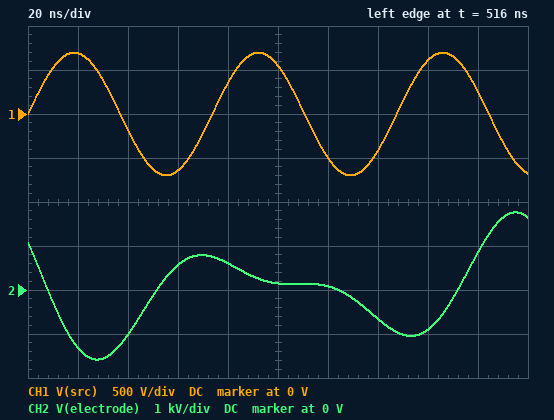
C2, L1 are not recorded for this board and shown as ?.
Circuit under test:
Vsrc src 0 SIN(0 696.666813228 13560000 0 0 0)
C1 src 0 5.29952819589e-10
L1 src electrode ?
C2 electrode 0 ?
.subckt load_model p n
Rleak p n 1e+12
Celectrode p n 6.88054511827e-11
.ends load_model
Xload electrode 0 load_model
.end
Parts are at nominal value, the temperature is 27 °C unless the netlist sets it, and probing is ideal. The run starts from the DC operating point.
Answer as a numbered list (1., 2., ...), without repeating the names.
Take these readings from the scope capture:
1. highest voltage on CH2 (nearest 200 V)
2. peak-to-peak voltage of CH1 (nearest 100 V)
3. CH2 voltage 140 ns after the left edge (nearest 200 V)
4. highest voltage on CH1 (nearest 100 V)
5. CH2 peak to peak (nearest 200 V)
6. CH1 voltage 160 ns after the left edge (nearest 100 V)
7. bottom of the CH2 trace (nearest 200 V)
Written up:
1. 1.8 kV
2. 1.4 kV
3. -600 V
4. 700 V
5. 3.4 kV
6. 600 V
7. -1.6 kV
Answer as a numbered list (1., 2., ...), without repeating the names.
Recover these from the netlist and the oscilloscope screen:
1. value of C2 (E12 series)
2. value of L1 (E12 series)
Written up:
1. 220 pF
2. 820 nH
